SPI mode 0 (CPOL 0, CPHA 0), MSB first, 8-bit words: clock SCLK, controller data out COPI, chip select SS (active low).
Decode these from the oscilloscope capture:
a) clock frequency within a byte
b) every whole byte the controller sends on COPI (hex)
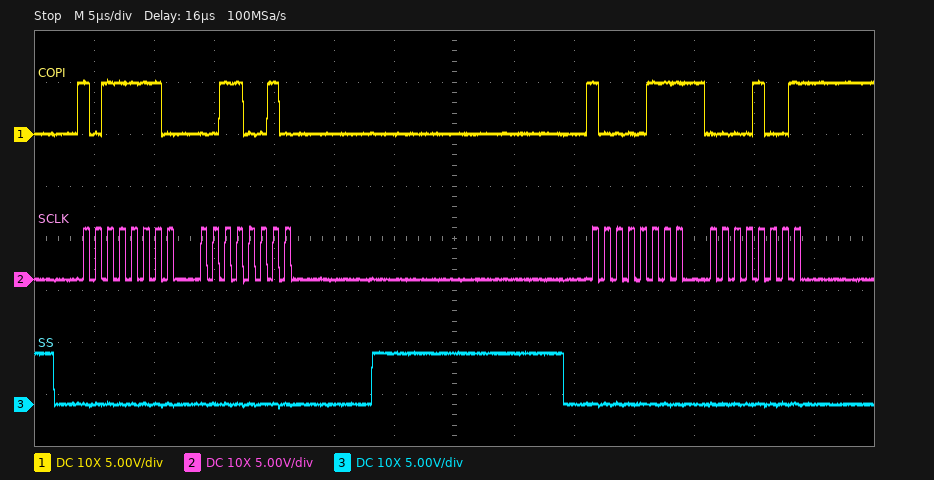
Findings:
1 MHz
BE 32 87 09
